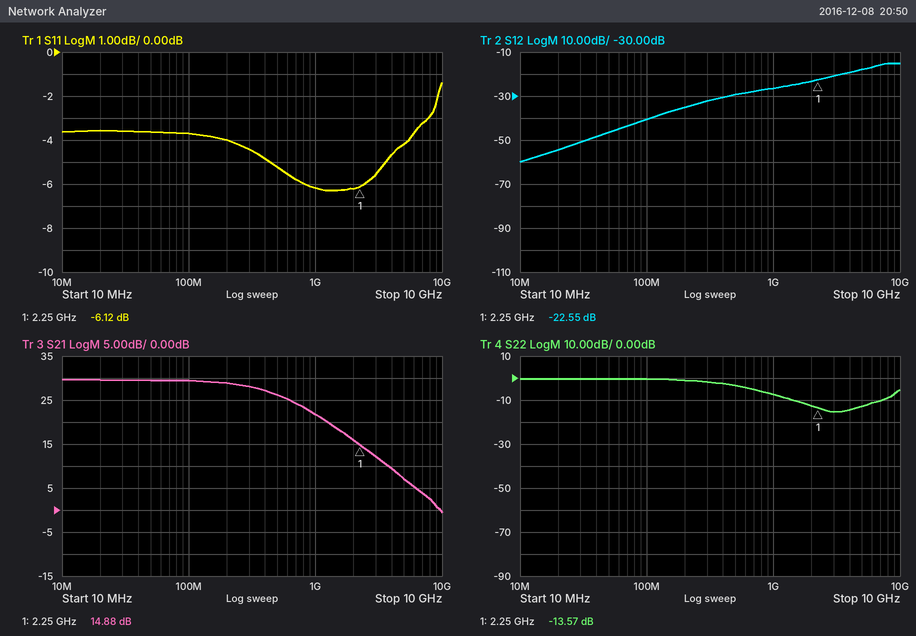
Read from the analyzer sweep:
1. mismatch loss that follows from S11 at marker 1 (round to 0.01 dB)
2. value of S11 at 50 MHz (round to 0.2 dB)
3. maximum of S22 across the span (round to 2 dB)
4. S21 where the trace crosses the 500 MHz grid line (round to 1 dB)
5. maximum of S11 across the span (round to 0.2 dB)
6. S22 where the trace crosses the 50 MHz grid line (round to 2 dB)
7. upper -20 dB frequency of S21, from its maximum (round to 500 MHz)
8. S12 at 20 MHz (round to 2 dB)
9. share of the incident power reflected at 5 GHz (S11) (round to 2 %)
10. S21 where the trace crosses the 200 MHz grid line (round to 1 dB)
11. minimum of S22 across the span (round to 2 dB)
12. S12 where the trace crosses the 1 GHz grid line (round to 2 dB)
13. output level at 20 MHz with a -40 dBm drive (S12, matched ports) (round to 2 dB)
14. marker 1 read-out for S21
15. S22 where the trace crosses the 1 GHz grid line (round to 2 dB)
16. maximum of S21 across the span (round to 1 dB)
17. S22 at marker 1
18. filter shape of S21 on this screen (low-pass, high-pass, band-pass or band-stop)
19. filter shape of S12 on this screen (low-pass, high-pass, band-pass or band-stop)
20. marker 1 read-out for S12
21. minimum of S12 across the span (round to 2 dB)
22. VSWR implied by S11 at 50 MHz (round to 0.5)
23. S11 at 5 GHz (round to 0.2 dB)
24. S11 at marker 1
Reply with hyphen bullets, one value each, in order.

- 1.22 dB
- -3.6 dB
- 0 dB
- 26 dB
- -1.4 dB
- 0 dB
- 4.0 GHz
- -54 dB
- 38 %
- 29 dB
- -16 dB
- -26 dB
- -94 dBm
- 14.88 dB
- -8 dB
- 30 dB
- -13.57 dB
- low-pass
- high-pass
- -22.55 dB
- -60 dB
- 5.0
- -4.2 dB
- -6.12 dB
